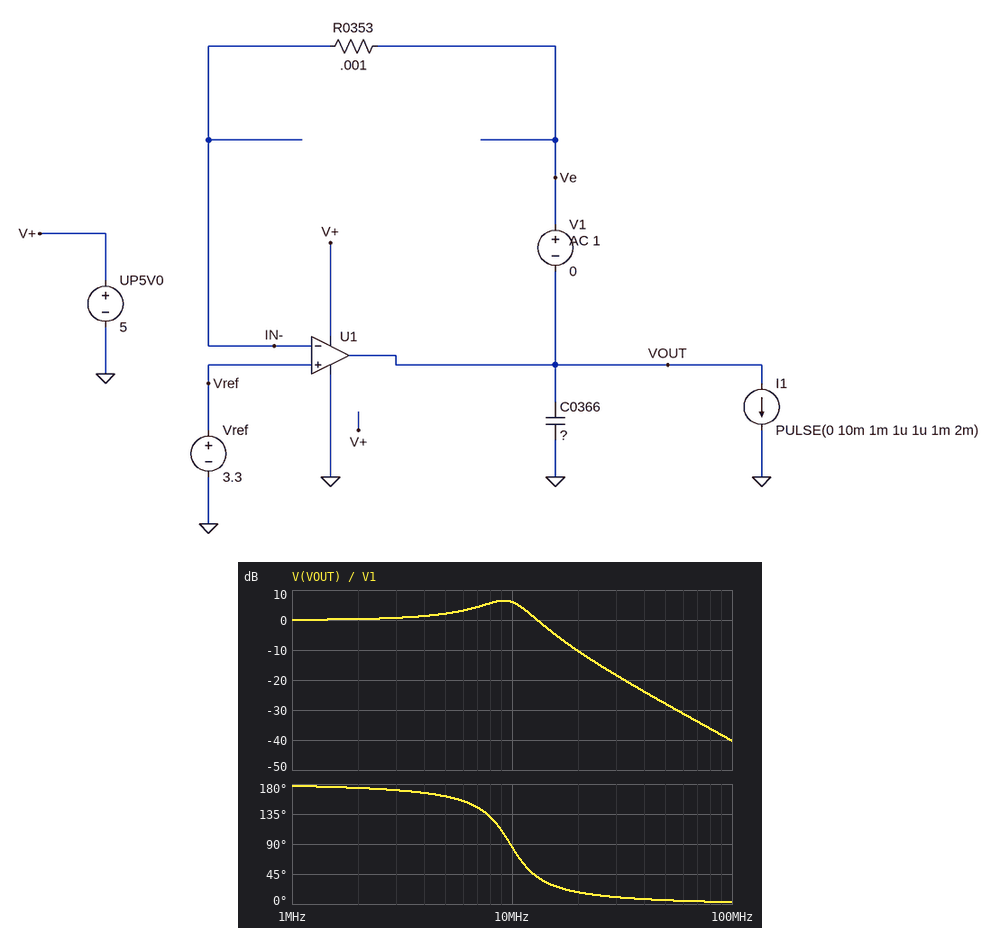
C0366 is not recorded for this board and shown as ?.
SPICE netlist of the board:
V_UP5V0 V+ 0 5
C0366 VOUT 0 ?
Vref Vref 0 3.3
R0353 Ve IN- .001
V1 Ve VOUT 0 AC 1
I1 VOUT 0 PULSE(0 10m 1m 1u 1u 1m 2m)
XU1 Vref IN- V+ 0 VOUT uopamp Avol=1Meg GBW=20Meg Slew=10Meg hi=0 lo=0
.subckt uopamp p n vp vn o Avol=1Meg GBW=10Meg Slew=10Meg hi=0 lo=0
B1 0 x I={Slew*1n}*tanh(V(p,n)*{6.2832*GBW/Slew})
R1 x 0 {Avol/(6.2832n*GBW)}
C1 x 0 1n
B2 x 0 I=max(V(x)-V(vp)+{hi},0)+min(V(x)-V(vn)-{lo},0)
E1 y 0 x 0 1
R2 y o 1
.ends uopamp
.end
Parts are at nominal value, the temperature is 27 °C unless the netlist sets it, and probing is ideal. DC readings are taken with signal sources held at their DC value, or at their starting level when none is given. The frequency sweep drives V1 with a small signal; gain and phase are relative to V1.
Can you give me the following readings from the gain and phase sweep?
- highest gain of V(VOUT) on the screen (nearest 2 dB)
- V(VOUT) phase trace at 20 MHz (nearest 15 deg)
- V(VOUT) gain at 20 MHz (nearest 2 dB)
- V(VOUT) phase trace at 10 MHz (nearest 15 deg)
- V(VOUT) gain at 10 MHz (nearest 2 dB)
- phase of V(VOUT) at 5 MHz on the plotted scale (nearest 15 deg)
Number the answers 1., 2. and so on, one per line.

1. 6 dB
2. 15 deg
3. -10 dB
4. 90 deg
5. 6 dB
6. 165 deg
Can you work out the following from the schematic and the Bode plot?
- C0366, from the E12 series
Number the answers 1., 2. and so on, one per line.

1. 33 nF
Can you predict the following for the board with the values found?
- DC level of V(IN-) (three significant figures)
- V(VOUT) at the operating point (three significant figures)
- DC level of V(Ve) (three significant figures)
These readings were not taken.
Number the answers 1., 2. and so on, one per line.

1. 3.30 V
2. 3.30 V
3. 3.30 V
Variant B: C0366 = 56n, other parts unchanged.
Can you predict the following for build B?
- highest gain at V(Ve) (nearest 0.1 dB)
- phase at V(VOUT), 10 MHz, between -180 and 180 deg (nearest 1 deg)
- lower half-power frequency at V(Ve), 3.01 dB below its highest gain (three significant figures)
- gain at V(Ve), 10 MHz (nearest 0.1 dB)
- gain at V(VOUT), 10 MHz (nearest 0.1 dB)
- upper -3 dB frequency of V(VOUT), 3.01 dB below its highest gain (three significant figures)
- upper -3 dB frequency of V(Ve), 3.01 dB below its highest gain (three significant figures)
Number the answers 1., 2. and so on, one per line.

1. 9.2 dB
2. 33 deg
3. 6.57 MHz
4. 6.1 dB
5. 0.8 dB
6. 8.59 MHz
7. 9.94 MHz
